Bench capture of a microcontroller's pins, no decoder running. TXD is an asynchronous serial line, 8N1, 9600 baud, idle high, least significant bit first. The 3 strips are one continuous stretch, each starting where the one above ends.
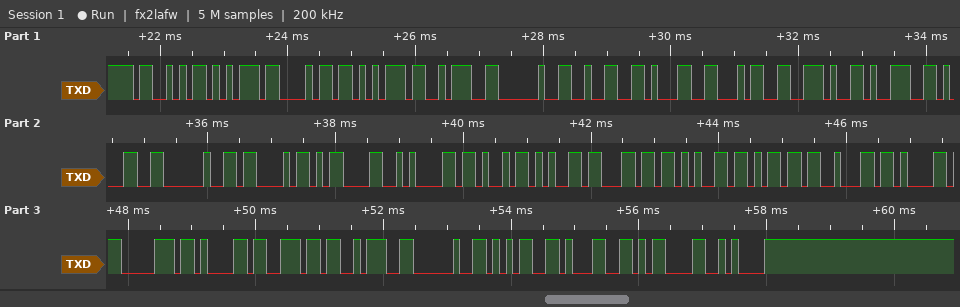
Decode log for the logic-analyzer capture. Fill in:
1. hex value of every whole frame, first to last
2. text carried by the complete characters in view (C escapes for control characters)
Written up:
0x53 0x75 0x68 0x75 0x3A 0x20 0x32 0x31 0x34 0x2E 0x39 0x31 0x20 0x43 0x0D 0x0A 0x4B 0x65 0x6C 0x65 0x6D 0x62 0x61 0x70 0x61 0x6E 0x3A 0x20 0x35 0x31 0x0D 0x0A
"Suhu: 214.91 C\r\nKelembapan: 51\r\n"
